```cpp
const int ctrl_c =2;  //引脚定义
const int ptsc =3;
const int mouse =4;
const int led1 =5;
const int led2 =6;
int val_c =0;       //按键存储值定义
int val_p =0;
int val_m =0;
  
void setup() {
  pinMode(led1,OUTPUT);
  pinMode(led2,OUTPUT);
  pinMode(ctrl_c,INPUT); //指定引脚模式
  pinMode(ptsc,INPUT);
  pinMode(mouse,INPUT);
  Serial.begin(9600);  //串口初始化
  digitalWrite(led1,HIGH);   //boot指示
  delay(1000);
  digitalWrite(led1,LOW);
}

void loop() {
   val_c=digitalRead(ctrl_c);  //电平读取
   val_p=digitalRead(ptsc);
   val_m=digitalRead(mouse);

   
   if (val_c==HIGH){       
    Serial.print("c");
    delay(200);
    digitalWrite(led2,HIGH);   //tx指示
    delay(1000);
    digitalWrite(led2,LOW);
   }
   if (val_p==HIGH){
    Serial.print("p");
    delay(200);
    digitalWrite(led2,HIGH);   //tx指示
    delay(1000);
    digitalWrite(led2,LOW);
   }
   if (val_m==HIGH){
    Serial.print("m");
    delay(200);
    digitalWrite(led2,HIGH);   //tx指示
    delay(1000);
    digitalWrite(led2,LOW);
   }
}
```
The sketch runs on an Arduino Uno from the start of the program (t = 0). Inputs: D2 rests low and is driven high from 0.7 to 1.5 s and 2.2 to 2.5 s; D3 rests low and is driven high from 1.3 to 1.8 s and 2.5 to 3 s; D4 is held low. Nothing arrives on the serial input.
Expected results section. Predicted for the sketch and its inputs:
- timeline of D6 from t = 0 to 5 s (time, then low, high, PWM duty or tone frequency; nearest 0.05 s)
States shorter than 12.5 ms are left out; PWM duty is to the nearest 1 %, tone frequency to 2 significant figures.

0 s low; 1.2 s high; 2.2 s low; 2.4 s high; 3.4 s low
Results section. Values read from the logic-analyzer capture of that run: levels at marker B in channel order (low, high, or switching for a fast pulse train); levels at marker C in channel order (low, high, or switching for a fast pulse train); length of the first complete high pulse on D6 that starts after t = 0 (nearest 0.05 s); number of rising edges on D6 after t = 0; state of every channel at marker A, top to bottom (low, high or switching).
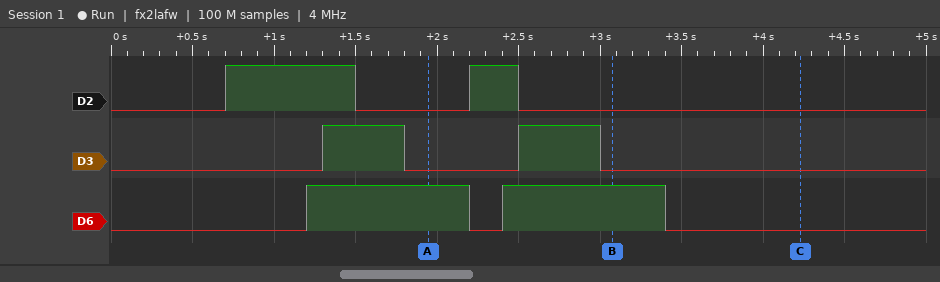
D2 low, D3 low, D6 high
D2 low, D3 low, D6 low
1.00 s
2
D2 low, D3 low, D6 high
